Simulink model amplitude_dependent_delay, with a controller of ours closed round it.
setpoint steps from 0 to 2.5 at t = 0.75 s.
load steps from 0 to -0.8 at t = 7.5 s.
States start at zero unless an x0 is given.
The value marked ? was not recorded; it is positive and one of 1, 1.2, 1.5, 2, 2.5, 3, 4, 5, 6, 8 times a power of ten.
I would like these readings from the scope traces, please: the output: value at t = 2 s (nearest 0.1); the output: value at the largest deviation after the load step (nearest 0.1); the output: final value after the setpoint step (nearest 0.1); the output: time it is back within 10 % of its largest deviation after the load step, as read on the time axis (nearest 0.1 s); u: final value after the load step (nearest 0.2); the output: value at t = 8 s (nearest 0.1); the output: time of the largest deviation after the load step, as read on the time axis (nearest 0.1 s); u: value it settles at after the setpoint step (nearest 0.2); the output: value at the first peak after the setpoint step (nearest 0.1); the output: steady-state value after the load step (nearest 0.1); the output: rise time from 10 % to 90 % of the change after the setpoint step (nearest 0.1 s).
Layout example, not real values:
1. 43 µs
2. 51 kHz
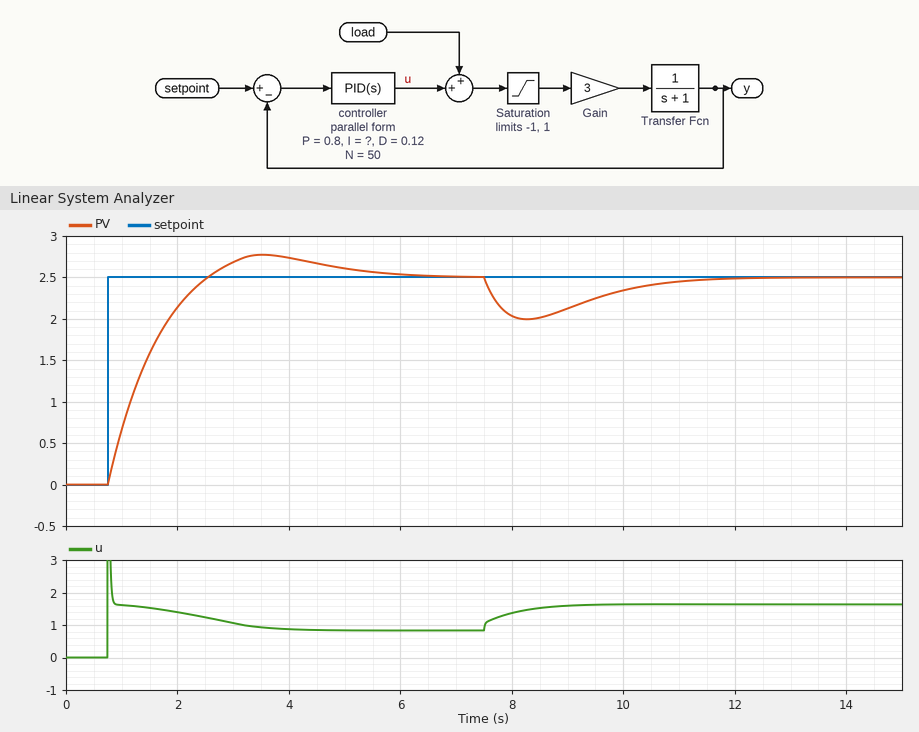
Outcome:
1. 2.1
2. 2.0
3. 2.5
4. 11.0 s
5. 1.6
6. 2.0
7. 8.3 s
8. 0.8
9. 2.8
10. 2.5
11. 1.3 s
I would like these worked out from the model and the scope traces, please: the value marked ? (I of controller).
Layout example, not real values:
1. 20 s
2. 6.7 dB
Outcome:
1. 0.8
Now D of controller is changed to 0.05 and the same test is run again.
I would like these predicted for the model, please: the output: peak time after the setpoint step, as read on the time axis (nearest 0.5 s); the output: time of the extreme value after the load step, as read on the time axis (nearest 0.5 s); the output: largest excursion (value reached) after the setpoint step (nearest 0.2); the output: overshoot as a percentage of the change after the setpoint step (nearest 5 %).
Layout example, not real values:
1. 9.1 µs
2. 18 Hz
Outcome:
1. 3.5 s
2. 8.0 s
3. 2.8
4. 10 %
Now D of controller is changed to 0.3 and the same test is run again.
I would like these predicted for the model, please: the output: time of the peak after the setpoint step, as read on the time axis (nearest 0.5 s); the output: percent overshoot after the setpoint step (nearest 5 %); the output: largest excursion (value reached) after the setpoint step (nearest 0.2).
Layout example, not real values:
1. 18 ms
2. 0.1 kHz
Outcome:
1. 3.5 s
2. 10 %
3. 2.8
